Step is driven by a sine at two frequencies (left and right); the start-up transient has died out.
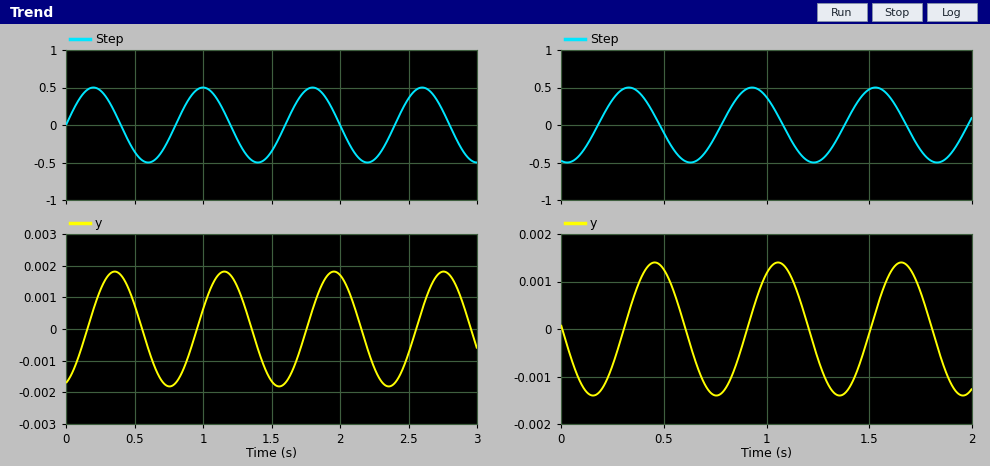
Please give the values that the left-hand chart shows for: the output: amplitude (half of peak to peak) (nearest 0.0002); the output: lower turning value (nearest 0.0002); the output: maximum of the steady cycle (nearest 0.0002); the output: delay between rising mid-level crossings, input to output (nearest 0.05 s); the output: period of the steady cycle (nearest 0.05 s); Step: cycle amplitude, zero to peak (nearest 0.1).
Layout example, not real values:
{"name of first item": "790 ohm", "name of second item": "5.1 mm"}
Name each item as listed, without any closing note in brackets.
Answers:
{"the output: amplitude (half of peak to peak)": "0.0018", "the output: lower turning value": "-0.0018", "the output: maximum of the steady cycle": "0.0018", "the output: delay between rising mid-level crossings, input to output": "0.15 s", "the output: period of the steady cycle": "0.80 s", "Step: cycle amplitude, zero to peak": "0.5"}
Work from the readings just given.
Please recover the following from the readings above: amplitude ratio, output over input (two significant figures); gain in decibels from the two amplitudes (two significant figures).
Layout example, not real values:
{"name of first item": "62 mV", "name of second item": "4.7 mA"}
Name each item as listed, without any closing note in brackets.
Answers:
{"amplitude ratio, output over input": "0.0036", "gain in decibels from the two amplitudes": "-49 dB"}
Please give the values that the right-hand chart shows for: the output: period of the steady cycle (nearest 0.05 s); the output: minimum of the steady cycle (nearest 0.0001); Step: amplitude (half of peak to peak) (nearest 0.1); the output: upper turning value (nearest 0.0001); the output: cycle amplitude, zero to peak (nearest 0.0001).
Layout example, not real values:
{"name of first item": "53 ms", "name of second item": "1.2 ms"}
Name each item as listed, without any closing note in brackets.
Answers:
{"the output: period of the steady cycle": "0.60 s", "the output: minimum of the steady cycle": "-0.0014", "Step: amplitude (half of peak to peak)": "0.5", "the output: upper turning value": "0.0014", "the output: cycle amplitude, zero to peak": "0.0014"}
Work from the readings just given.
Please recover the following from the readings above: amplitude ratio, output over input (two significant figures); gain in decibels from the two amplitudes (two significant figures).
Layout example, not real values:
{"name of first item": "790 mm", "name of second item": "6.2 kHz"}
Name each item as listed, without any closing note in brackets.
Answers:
{"amplitude ratio, output over input": "0.0028", "gain in decibels from the two amplitudes": "-51 dB"}
